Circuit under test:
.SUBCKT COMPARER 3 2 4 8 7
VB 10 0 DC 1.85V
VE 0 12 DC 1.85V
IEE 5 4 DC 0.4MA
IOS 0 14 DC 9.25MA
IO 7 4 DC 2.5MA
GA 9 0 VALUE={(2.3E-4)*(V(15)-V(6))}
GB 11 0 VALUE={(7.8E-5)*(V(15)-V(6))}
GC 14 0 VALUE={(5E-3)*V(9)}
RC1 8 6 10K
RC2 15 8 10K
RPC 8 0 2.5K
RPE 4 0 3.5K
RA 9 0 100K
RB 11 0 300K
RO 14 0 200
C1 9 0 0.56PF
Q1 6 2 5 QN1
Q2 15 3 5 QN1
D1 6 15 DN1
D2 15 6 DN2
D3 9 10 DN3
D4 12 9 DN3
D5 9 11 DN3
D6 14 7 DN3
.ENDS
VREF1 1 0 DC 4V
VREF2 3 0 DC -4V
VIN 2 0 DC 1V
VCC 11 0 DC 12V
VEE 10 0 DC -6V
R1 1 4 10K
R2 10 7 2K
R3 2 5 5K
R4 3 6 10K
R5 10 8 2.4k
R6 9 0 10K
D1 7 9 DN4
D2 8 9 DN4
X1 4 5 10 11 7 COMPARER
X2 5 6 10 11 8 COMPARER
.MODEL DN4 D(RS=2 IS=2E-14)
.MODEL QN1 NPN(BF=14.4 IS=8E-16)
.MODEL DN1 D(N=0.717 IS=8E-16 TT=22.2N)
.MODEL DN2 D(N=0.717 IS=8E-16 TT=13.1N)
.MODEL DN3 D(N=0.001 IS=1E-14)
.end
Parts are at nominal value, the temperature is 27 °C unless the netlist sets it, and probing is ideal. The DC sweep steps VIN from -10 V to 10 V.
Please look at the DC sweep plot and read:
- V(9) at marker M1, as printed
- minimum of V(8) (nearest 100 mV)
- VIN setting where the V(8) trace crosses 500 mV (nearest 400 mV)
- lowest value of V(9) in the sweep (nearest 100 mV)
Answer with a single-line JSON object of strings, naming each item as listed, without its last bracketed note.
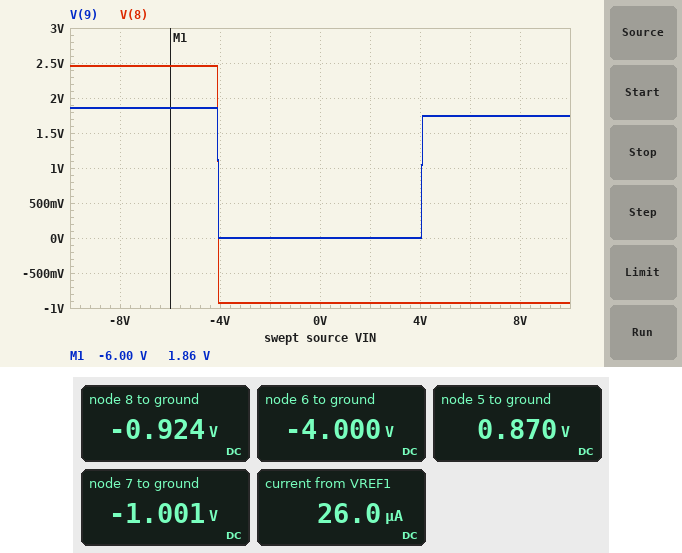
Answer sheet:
{"V(9) at marker M1, as printed": "1.86 V", "minimum of V(8)": "-900 mV", "VIN setting where the V(8) trace crosses 500 mV": "-4.0 V", "lowest value of V(9) in the sweep": "0 V"}
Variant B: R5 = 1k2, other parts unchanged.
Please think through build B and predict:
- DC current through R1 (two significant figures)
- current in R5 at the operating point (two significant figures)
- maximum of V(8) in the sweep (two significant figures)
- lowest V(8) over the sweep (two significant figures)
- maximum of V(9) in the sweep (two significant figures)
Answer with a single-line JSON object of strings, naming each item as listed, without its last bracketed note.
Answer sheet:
{"DC current through R1": "26 µA", "current in R5 at the operating point": "3.9 mA", "maximum of V(8) in the sweep": "1.9 V", "lowest V(8) over the sweep": "-1.3 V", "maximum of V(9) in the sweep": "1.7 V"}
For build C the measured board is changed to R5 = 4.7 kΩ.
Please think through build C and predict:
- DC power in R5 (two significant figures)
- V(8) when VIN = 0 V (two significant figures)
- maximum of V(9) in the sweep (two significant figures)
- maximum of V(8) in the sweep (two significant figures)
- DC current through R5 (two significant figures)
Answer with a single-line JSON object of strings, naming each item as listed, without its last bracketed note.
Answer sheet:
{"DC power in R5": "5.9 mW", "V(8) when VIN = 0 V": "-730 mV", "maximum of V(9) in the sweep": "2.2 V", "maximum of V(8) in the sweep": "2.8 V", "DC current through R5": "1.1 mA"}
